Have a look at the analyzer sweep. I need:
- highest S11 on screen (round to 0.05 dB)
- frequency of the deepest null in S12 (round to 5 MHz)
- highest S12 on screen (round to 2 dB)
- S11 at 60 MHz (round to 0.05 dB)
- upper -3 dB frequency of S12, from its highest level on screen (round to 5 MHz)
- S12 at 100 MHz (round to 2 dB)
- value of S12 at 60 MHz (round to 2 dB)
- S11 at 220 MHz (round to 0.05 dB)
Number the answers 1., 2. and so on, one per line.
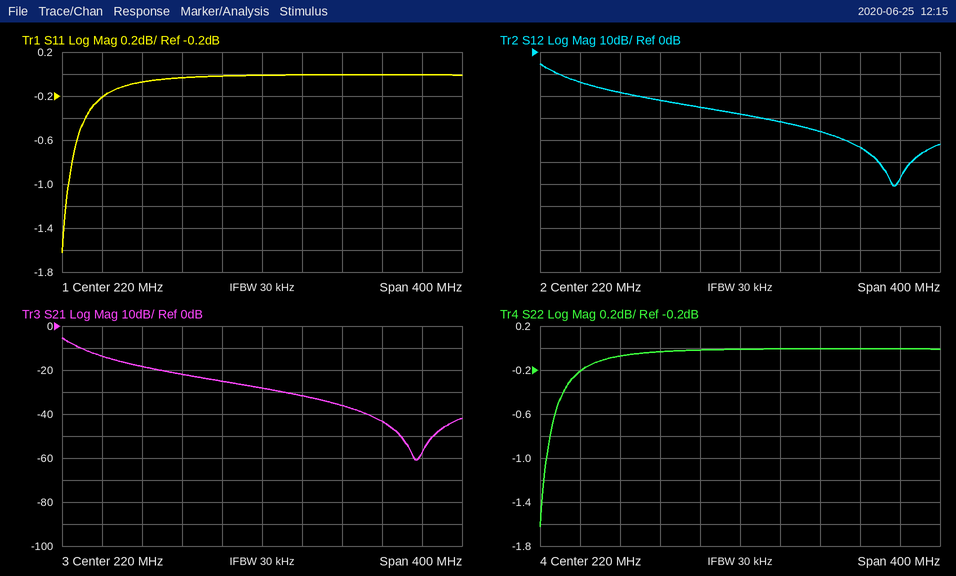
1. 0.00 dB
2. 375 MHz
3. -6 dB
4. -0.20 dB
5. 30 MHz
6. -18 dB
7. -14 dB
8. 0.00 dB
